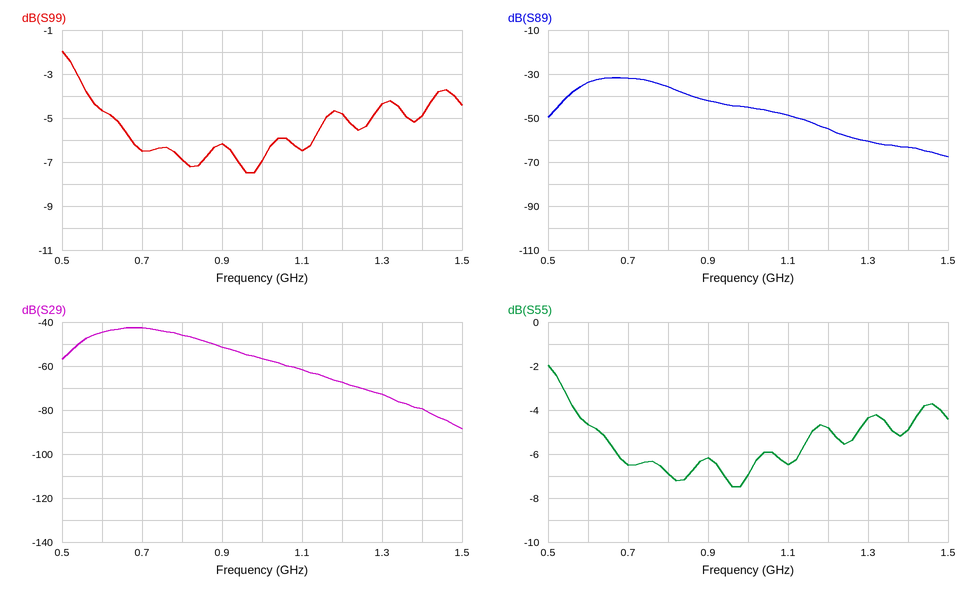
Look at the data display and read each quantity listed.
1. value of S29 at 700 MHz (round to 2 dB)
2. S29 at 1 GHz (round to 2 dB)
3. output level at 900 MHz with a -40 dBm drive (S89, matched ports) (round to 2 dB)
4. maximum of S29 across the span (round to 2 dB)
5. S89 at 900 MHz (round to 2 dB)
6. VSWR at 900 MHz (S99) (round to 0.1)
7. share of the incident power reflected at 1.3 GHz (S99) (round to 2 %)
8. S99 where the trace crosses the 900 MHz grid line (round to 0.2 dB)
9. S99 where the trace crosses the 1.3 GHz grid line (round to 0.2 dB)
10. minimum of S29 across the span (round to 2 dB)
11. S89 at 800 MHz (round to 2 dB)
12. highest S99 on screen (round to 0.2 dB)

-42 dB
-56 dB
-82 dBm
-42 dB
-42 dB
2.9
36 %
-6.2 dB
-4.4 dB
-88 dB
-36 dB
-2.0 dB
